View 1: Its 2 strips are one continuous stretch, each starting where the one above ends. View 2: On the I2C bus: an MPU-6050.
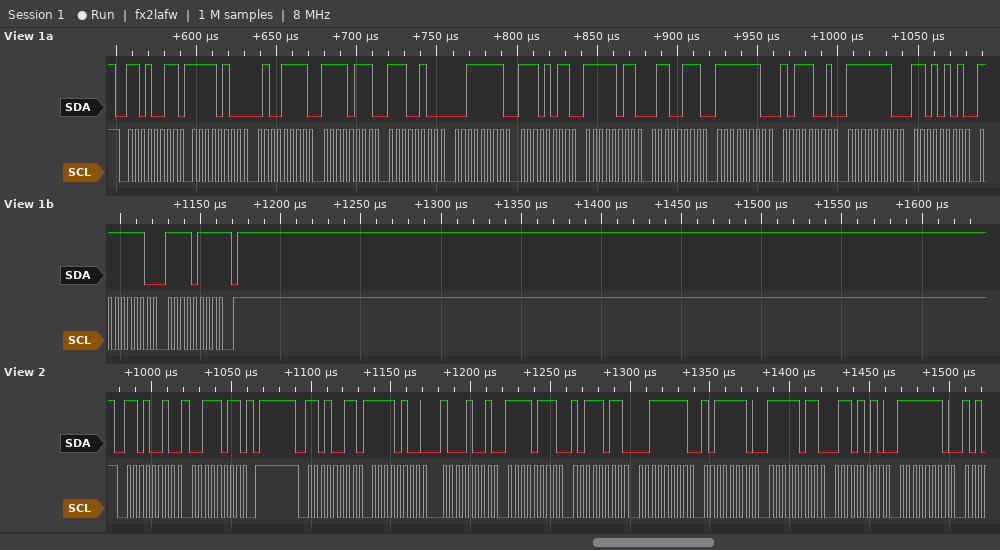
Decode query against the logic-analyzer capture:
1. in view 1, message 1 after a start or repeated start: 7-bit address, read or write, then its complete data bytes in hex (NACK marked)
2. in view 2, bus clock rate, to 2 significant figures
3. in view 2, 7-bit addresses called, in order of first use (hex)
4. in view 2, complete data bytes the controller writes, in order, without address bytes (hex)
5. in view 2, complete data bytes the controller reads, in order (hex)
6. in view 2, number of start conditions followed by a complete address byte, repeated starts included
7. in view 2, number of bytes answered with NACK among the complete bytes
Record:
0x69 read: F4 4F F7 E4 3F EB FB 67 FE B9 FE D5 FE F7 NACK
250 kHz
0x69
3B
F4 89 F7 BB 3F BE FB 6A FE
2
0
